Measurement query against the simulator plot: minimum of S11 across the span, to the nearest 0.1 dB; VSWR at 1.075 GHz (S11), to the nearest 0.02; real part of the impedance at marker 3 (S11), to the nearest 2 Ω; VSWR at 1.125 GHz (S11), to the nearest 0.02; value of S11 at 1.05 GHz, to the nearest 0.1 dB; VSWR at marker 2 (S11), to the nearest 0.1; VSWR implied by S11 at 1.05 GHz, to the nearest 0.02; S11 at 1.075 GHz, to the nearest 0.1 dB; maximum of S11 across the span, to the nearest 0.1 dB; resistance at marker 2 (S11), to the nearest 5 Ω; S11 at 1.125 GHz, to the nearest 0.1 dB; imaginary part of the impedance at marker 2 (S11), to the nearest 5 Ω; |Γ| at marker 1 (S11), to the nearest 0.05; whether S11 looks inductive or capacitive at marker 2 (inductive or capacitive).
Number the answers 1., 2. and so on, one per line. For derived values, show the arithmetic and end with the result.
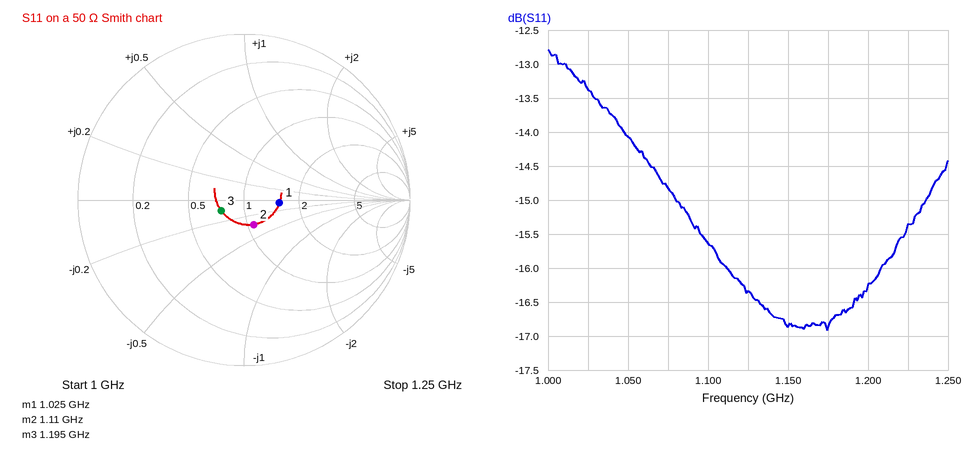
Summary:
1. -16.9 dB
2. |Γ| = 10^(-14.8/20) = 0.1820; VSWR = (1 + 0.1820)/(1 − 0.1820) ≈ 1.44
3. 38 Ω
4. |Γ| = 10^(-16.3/20) = 0.1531; VSWR = (1 + 0.1531)/(1 − 0.1531) ≈ 1.36
5. -14.1 dB
6. 1.4
7. |Γ| = 10^(-14.1/20) = 0.1972; VSWR = (1 + 0.1972)/(1 − 0.1972) ≈ 1.49, so 1.50 to the nearest 0.02
8. -14.8 dB
9. -12.8 dB
10. 55 Ω
11. -16.3 dB
12. -15 Ω
13. 0.20
14. capacitive
